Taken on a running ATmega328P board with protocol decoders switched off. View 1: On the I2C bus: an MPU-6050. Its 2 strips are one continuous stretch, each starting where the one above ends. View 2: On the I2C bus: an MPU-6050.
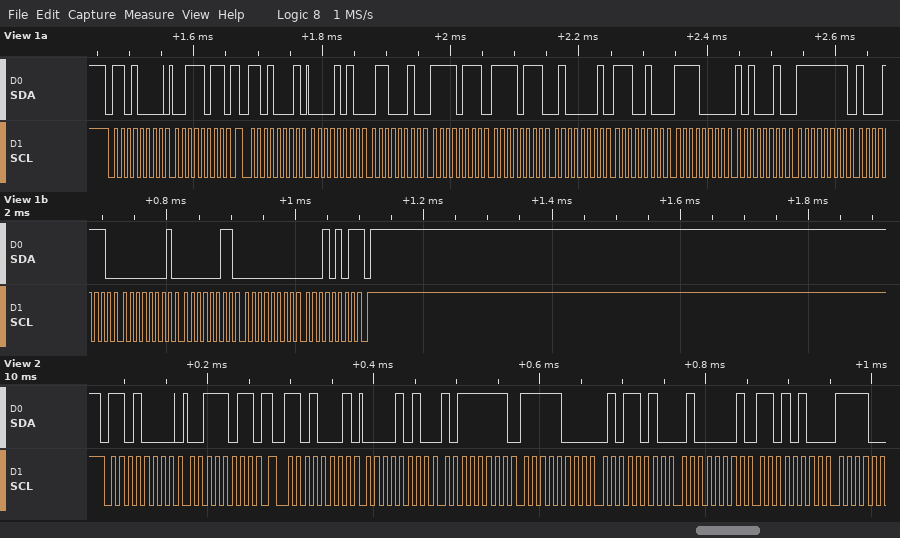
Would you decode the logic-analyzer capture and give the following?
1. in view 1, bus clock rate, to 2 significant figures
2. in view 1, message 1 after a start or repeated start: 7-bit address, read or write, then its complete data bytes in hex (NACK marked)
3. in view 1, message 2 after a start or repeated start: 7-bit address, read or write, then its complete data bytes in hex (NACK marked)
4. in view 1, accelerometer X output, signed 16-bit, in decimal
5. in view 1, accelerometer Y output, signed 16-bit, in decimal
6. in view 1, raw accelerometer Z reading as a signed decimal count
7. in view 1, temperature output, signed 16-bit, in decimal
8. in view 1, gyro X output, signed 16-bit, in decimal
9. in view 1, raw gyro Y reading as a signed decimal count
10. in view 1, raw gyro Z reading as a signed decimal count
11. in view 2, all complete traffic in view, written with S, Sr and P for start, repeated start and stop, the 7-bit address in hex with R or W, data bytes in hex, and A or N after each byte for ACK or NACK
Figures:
100 kHz
0x68 write: 3B
0x68 read: 0A 62 F7 F7 41 E4 F0 A2 FF 8E 01 03 00 15 NACK
2658
-2057
16868
-3934
-114
259
21
S 68W A 3B A Sr 68R A 0A A BF A F8 A 5A A 41 A D4 A
